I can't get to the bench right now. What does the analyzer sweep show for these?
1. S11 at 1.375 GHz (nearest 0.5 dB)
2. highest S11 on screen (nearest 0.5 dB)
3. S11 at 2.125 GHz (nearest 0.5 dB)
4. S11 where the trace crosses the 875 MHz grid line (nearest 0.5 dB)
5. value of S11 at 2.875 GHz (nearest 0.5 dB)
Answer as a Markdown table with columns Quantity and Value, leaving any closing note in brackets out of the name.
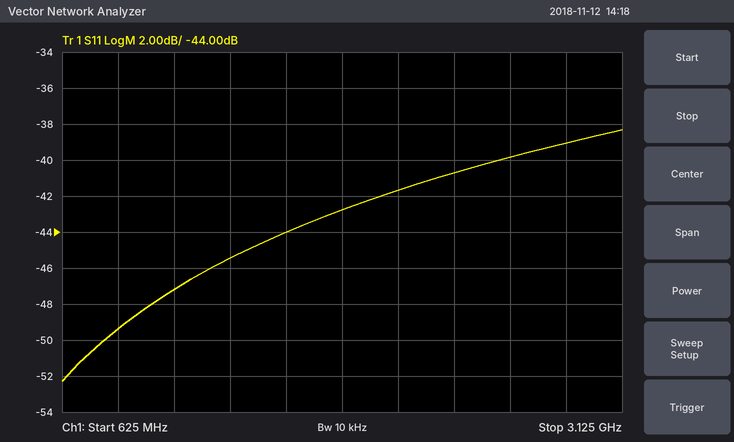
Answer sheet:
| Quantity | Value |
|---|---|
| S11 at 1.375 GHz | -45.5 dB |
| highest S11 on screen | -38.5 dB |
| S11 at 2.125 GHz | -41.5 dB |
| S11 where the trace crosses the 875 MHz grid line | -49.5 dB |
| value of S11 at 2.875 GHz | -39.0 dB |
